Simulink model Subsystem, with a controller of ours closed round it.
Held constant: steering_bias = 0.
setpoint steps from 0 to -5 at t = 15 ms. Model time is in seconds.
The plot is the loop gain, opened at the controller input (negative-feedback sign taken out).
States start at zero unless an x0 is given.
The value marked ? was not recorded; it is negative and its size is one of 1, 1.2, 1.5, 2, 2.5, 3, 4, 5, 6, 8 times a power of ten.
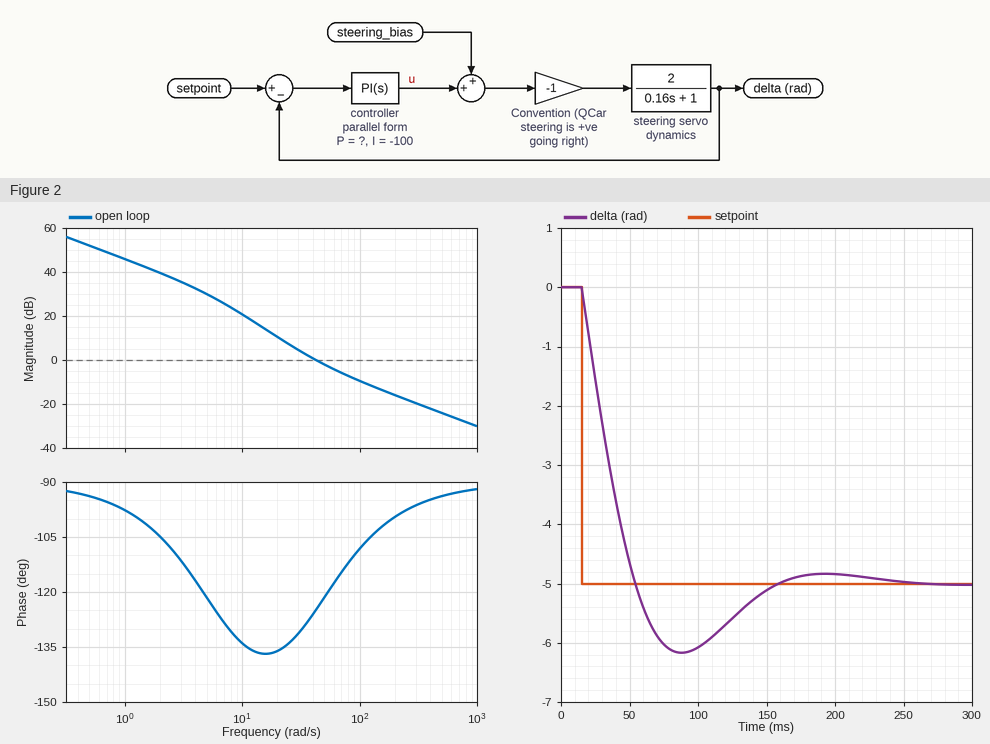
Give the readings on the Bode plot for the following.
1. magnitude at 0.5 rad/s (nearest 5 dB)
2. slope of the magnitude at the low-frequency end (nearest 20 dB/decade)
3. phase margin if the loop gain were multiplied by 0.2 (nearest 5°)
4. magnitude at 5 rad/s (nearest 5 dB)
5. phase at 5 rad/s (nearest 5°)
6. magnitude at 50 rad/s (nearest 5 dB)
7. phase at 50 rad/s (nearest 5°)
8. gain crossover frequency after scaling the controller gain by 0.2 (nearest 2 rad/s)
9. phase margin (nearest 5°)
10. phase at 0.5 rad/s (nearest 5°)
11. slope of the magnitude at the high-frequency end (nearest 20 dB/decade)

50 dB
-20 dB/decade
45°
30 dB
-120°
0 dB
-120°
16 rad/s
55°
-95°
-20 dB/decade
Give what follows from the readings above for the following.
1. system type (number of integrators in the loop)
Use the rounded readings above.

1
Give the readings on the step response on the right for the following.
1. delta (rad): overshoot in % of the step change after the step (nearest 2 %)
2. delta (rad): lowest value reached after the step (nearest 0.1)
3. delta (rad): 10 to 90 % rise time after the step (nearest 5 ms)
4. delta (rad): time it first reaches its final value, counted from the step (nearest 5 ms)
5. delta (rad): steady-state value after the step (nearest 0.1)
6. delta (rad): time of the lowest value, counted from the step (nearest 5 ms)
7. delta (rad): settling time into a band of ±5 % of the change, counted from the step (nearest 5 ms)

24 %
-6.2
30 ms
40 ms
-5.0
75 ms
125 ms
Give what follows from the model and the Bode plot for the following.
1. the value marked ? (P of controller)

-2.5
